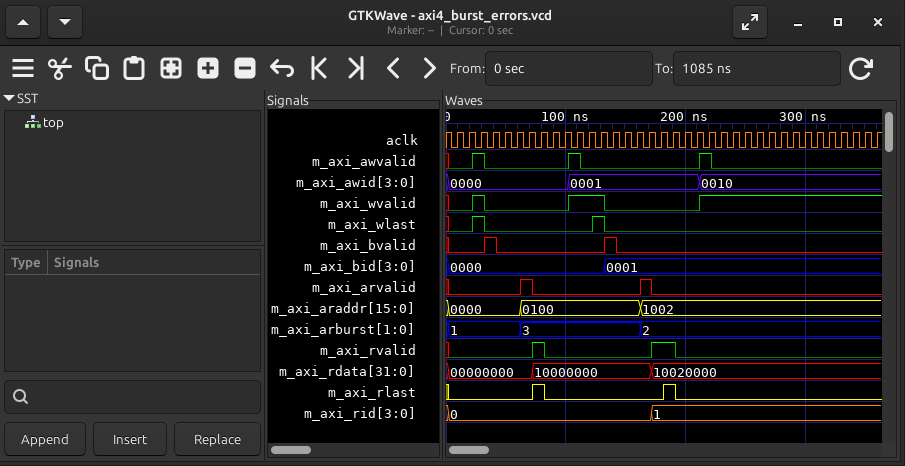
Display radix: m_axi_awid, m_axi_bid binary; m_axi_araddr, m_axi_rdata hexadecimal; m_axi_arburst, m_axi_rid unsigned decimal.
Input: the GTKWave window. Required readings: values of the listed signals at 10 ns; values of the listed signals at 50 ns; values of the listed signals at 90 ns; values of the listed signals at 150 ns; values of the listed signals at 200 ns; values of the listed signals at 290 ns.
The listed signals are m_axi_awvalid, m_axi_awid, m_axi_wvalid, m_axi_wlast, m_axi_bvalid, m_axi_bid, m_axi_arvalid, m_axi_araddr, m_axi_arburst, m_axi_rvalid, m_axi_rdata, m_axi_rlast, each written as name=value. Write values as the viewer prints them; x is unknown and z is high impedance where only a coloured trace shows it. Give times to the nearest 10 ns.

m_axi_awvalid=0, m_axi_awid=0000, m_axi_wvalid=0, m_axi_wlast=0, m_axi_bvalid=0, m_axi_bid=0000, m_axi_arvalid=0, m_axi_araddr=0000, m_axi_arburst=1, m_axi_rvalid=0, m_axi_rdata=00000000, m_axi_rlast=0
m_axi_awvalid=0, m_axi_awid=0000, m_axi_wvalid=0, m_axi_wlast=0, m_axi_bvalid=0, m_axi_bid=0000, m_axi_arvalid=0, m_axi_araddr=0000, m_axi_arburst=1, m_axi_rvalid=0, m_axi_rdata=00000000, m_axi_rlast=0
m_axi_awvalid=0, m_axi_awid=0000, m_axi_wvalid=0, m_axi_wlast=0, m_axi_bvalid=0, m_axi_bid=0000, m_axi_arvalid=0, m_axi_araddr=0100, m_axi_arburst=3, m_axi_rvalid=0, m_axi_rdata=10000000, m_axi_rlast=0
m_axi_awvalid=0, m_axi_awid=0001, m_axi_wvalid=0, m_axi_wlast=0, m_axi_bvalid=0, m_axi_bid=0001, m_axi_arvalid=0, m_axi_araddr=0100, m_axi_arburst=3, m_axi_rvalid=0, m_axi_rdata=10000000, m_axi_rlast=0
m_axi_awvalid=0, m_axi_awid=0001, m_axi_wvalid=0, m_axi_wlast=0, m_axi_bvalid=0, m_axi_bid=0001, m_axi_arvalid=0, m_axi_araddr=1002, m_axi_arburst=2, m_axi_rvalid=0, m_axi_rdata=10020000, m_axi_rlast=0
m_axi_awvalid=0, m_axi_awid=0010, m_axi_wvalid=1, m_axi_wlast=0, m_axi_bvalid=0, m_axi_bid=0001, m_axi_arvalid=0, m_axi_araddr=1002, m_axi_arburst=2, m_axi_rvalid=0, m_axi_rdata=10020000, m_axi_rlast=0
